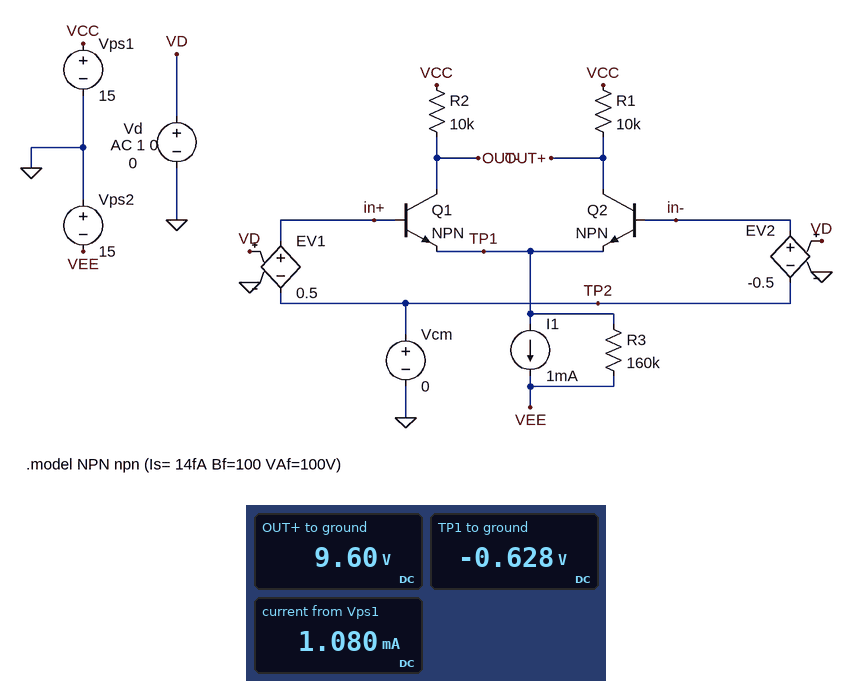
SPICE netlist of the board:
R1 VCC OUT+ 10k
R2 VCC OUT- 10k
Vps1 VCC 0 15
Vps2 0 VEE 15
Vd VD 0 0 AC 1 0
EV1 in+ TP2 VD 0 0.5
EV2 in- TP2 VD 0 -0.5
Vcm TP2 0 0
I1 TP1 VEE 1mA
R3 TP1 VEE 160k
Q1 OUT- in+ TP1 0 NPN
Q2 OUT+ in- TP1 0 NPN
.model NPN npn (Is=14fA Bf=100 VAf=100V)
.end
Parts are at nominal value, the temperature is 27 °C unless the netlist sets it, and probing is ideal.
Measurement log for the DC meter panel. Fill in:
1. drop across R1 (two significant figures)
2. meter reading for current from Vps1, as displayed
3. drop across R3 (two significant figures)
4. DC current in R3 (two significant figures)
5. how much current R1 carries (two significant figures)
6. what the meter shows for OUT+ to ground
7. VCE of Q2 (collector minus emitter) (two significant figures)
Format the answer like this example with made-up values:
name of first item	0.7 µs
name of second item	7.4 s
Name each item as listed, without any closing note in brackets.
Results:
drop across R1	5.4 V
meter reading for current from Vps1, as displayed	1.080 mA
drop across R3	14 V
DC current in R3	90 µA
how much current R1 carries	540 µA
what the meter shows for OUT+ to ground	9.60 V
VCE of Q2 (collector minus emitter)	10 V
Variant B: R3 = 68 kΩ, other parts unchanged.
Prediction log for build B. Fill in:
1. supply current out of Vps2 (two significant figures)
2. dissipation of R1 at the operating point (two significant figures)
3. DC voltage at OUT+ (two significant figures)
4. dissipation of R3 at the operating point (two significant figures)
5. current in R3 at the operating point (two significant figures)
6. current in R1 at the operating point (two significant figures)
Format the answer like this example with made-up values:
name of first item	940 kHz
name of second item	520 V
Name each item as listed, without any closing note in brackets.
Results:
supply current out of Vps2	1.2 mA
dissipation of R1 at the operating point	3.6 mW
DC voltage at OUT+	9.0 V
dissipation of R3 at the operating point	3.0 mW
current in R3 at the operating point	210 µA
current in R1 at the operating point	600 µA
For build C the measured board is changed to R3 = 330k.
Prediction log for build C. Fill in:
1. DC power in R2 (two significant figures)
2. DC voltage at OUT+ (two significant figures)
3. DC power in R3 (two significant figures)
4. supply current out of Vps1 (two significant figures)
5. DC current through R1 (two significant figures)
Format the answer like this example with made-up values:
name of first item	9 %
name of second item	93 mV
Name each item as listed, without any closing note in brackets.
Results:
DC power in R2	2.7 mW
DC voltage at OUT+	9.8 V
DC power in R3	630 µW
supply current out of Vps1	1.0 mA
DC current through R1	520 µA
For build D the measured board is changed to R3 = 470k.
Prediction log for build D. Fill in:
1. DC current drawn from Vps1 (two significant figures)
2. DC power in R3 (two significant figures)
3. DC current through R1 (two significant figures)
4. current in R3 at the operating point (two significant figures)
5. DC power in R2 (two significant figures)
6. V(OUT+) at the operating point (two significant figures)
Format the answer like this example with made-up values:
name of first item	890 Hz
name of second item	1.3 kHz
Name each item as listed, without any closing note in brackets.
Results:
DC current drawn from Vps1	1.0 mA
DC power in R3	440 µW
DC current through R1	510 µA
current in R3 at the operating point	31 µA
DC power in R2	2.6 mW
V(OUT+) at the operating point	9.9 V
